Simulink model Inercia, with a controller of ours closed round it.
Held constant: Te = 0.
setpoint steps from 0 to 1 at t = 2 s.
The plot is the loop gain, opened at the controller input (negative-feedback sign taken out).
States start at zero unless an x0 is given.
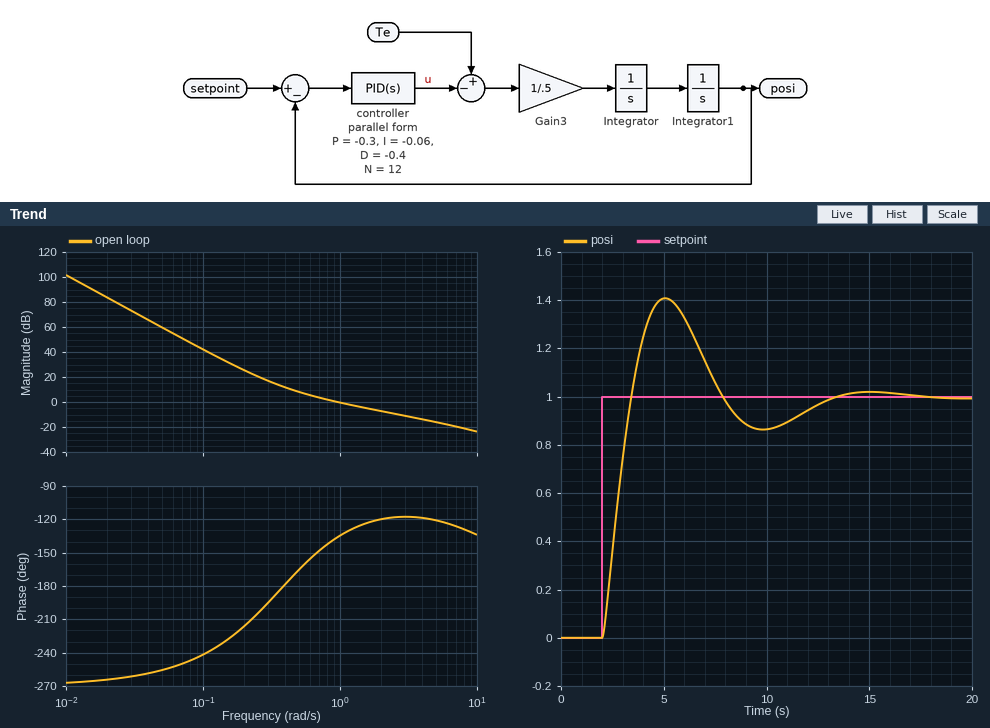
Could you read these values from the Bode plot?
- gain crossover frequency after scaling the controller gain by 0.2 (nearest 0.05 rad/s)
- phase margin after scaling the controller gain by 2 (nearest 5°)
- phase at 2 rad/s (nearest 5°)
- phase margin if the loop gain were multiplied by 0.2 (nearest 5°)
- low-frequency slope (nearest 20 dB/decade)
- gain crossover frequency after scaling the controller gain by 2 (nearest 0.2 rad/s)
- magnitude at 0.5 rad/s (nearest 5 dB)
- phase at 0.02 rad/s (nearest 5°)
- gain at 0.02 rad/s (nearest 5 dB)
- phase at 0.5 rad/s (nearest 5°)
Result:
0.35 rad/s
60°
-120°
-5°
-60 dB/decade
1.8 rad/s
10 dB
-265°
85 dB
-165°
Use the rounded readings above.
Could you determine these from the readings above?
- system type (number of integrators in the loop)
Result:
3
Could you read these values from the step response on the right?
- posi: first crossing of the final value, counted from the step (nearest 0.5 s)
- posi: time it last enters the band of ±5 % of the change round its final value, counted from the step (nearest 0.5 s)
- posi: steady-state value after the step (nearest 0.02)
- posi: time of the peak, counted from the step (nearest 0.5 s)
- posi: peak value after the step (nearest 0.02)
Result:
1.5 s
10.0 s
1.00
3.0 s
1.40
